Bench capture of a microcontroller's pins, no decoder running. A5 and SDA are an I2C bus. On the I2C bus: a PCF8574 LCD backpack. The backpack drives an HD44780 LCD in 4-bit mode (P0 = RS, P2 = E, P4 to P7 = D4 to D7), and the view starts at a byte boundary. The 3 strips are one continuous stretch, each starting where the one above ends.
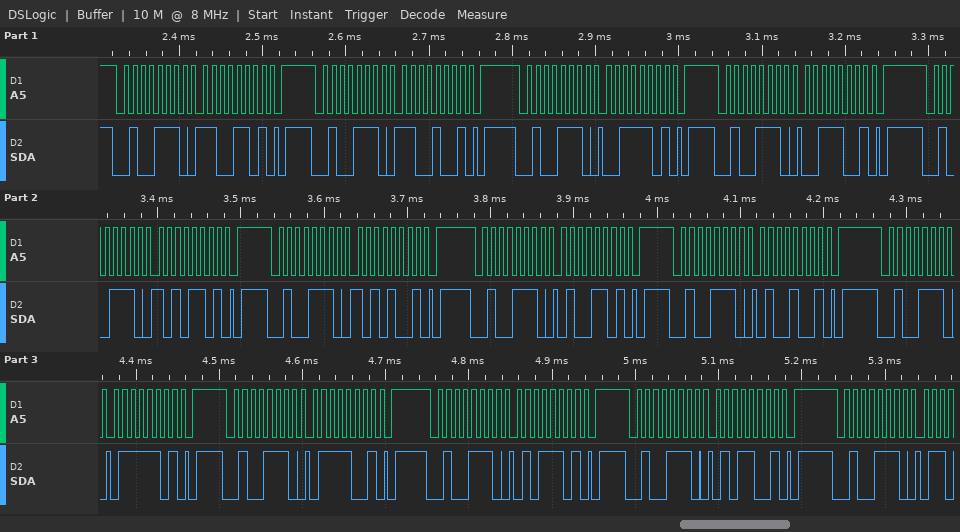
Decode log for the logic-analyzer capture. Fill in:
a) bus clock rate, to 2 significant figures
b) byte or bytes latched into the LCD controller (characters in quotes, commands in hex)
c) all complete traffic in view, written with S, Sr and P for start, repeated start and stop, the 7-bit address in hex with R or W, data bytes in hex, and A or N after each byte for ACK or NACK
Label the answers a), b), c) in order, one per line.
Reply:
a) 100 kHz
b) data 0xC3 data 0xA4 'u'
c) S 27W A CD A P S 27W A C9 A P S 27W A 3D A P S 27W A 39 A P S 27W A AD A P S 27W A A9 A P S 27W A 4D A P S 27W A 49 A P S 27W A 7D A P S 27W A 79 A P S 27W A 5D A P S 27W A 59 A P S 27W A
